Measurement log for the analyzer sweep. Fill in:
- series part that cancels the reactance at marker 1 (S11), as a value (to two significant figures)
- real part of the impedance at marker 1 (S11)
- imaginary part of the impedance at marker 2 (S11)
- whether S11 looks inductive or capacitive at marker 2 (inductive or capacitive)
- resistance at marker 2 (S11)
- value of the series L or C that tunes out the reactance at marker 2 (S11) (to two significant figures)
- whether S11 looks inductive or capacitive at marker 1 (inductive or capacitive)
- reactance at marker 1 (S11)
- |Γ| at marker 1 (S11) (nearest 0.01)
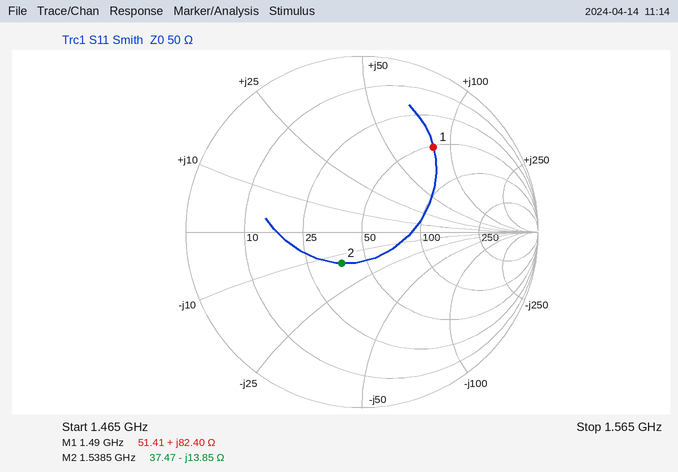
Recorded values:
1.3 pF
51.41 Ω
-13.85 Ω
capacitive
37.47 Ω
1.4 nH
inductive
+82.40 Ω
0.63
